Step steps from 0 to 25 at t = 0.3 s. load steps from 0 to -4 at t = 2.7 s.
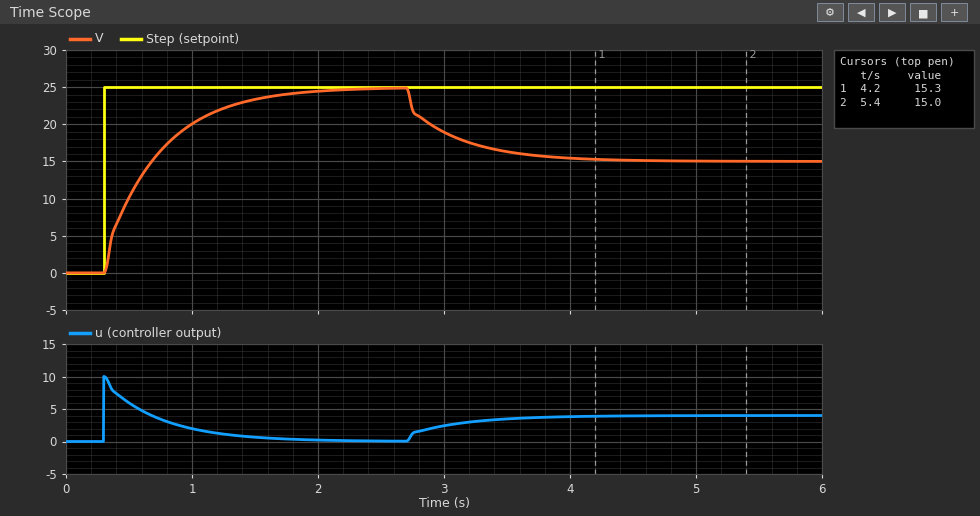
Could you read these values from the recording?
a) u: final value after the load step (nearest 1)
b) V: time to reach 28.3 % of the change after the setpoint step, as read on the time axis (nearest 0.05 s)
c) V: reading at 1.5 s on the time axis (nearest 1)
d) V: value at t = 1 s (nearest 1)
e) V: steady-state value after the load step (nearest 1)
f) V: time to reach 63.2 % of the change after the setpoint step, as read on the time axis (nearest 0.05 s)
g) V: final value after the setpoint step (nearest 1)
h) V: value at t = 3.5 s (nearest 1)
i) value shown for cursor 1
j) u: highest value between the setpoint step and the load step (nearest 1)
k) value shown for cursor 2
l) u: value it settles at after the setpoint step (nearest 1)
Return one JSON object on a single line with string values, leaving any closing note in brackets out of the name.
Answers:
{"u: final value after the load step": "4", "V: time to reach 28.3 % of the change after the setpoint step, as read on the time axis": "0.40 s", "V: reading at 1.5 s on the time axis": "23", "V: value at t = 1 s": "20", "V: steady-state value after the load step": "15", "V: time to reach 63.2 % of the change after the setpoint step, as read on the time axis": "0.70 s", "V: final value after the setpoint step": "25", "V: value at t = 3.5 s": "16", "value shown for cursor 1": "15.3", "u: highest value between the setpoint step and the load step": "10", "value shown for cursor 2": "15.0", "u: value it settles at after the setpoint step": "0"}
